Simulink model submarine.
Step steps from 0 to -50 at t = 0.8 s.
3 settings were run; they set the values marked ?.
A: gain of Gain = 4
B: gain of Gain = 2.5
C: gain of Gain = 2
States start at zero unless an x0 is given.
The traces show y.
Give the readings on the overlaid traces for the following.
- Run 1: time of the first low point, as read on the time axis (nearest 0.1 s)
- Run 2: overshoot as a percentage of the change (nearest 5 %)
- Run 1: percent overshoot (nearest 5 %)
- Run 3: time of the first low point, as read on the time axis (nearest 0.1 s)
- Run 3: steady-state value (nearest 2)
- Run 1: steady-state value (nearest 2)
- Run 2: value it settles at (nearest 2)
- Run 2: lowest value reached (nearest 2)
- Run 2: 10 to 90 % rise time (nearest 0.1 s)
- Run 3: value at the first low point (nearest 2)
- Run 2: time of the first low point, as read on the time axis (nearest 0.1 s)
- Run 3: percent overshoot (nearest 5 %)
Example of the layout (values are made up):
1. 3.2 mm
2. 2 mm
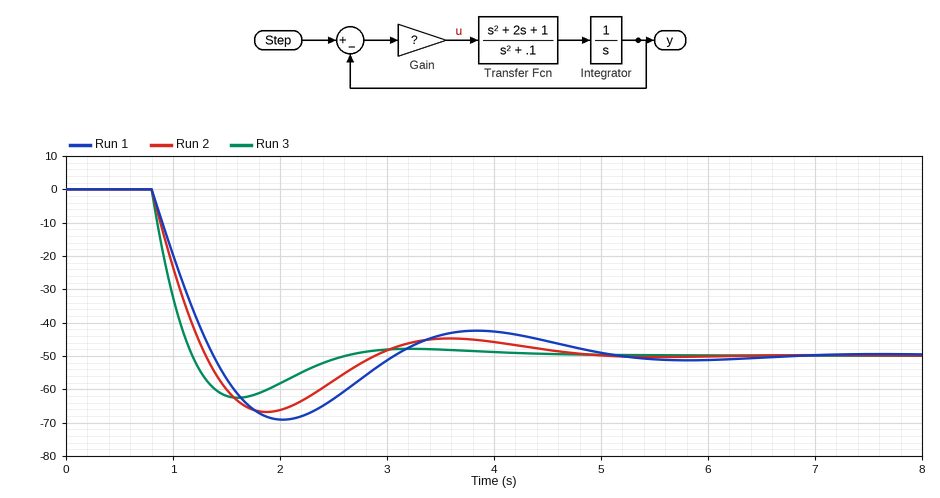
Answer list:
1. 2.0 s
2. 35 %
3. 40 %
4. 1.6 s
5. -50
6. -50
7. -50
8. -66
9. 0.4 s
10. -62
11. 1.9 s
12. 25 %
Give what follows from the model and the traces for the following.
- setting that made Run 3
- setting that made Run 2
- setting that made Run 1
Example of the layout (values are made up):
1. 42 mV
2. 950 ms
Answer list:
1. A
2. B
3. C
